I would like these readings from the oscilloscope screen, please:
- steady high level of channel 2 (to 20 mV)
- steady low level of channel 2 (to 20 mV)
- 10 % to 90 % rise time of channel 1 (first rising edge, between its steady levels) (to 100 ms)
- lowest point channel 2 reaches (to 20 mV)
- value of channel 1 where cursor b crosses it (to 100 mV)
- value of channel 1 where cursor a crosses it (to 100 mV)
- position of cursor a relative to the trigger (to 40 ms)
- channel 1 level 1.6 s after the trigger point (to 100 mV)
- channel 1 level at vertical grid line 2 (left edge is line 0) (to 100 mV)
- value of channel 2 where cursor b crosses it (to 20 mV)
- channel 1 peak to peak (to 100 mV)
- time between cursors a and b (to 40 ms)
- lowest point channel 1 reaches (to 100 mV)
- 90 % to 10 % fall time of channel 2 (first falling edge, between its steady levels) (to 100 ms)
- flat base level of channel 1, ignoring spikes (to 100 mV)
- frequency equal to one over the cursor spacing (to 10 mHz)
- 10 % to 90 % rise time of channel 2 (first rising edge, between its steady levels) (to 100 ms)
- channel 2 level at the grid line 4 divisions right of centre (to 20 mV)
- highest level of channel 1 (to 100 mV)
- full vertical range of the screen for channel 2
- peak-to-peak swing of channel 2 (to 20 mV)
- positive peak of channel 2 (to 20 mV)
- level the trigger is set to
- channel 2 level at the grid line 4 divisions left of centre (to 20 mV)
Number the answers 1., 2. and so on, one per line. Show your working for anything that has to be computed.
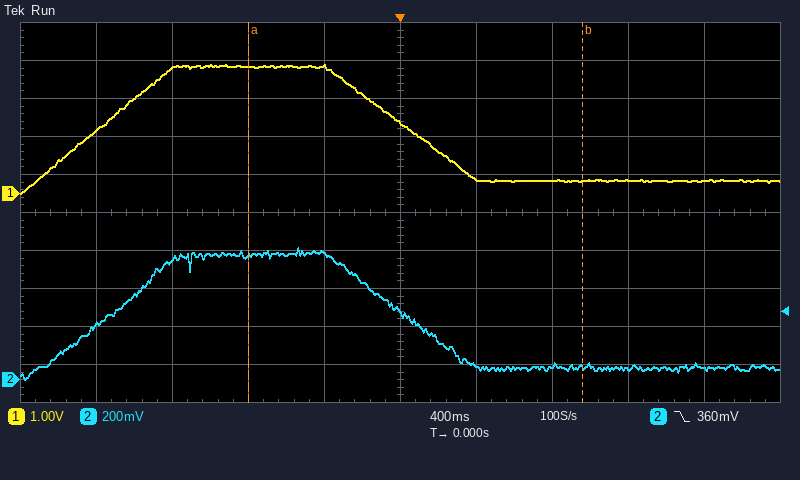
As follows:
1. 660 mV
2. 60 mV
3. 600 ms
4. 0 mV
5. 300 mV
6. 3.3 V
7. -800 ms
8. 300 mV
9. 3.3 V
10. 60 mV
11. 3.4 V − (0.0 V) = 3.4 V
12. 1.76 s
13. 0.0 V
14. 600 ms
15. 300 mV
16. 1 / 1.76 s ≈ 570 mHz
17. 600 ms
18. 60 mV
19. 3.4 V
20. 2 V
21. 700 mV − (0 mV) = 700 mV
22. 700 mV
23. 360 mV
24. 280 mV
